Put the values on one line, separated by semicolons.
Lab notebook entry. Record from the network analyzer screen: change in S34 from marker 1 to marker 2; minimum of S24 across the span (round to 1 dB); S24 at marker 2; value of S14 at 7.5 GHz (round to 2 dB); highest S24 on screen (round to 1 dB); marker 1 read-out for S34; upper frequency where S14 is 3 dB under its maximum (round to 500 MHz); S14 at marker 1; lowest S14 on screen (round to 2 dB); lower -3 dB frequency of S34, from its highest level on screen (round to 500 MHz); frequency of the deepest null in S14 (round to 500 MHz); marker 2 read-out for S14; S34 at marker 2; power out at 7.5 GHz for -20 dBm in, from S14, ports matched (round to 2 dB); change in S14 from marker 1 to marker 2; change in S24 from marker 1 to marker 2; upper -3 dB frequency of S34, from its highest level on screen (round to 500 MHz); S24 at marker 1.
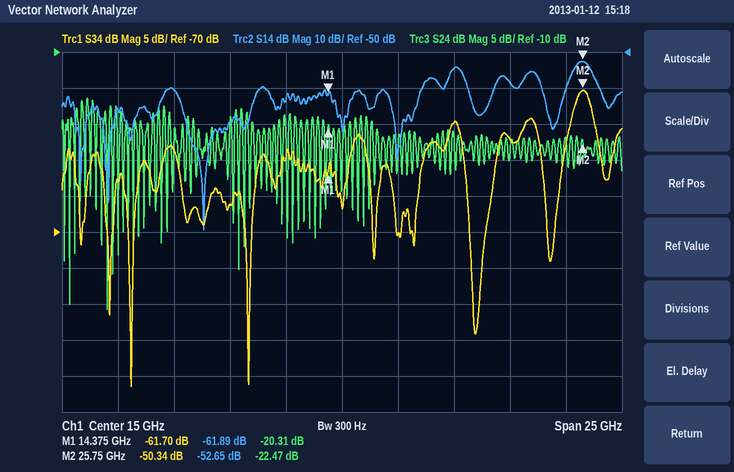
11.36 dB; -46 dB; -22.47 dB; -60 dB; -16 dB; -61.70 dB; 26.0 GHz; -61.89 dB; -100 dB; 25.5 GHz; 9.0 GHz; -52.65 dB; -50.34 dB; -80 dBm; 9.24 dB; -2.16 dB; 26.0 GHz; -20.31 dB
